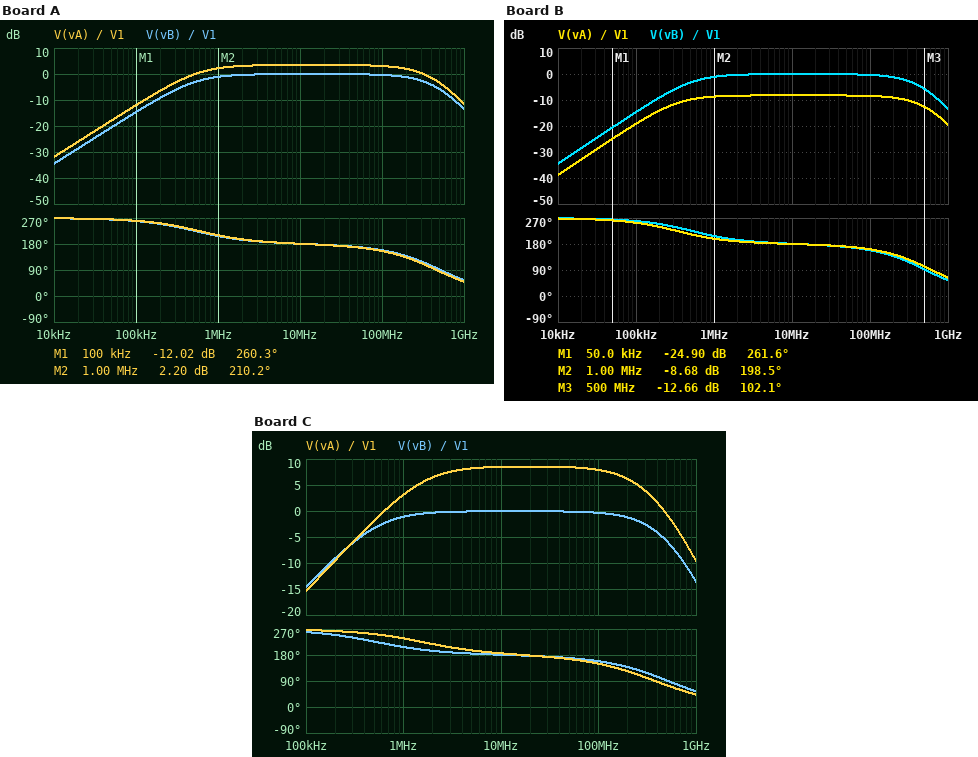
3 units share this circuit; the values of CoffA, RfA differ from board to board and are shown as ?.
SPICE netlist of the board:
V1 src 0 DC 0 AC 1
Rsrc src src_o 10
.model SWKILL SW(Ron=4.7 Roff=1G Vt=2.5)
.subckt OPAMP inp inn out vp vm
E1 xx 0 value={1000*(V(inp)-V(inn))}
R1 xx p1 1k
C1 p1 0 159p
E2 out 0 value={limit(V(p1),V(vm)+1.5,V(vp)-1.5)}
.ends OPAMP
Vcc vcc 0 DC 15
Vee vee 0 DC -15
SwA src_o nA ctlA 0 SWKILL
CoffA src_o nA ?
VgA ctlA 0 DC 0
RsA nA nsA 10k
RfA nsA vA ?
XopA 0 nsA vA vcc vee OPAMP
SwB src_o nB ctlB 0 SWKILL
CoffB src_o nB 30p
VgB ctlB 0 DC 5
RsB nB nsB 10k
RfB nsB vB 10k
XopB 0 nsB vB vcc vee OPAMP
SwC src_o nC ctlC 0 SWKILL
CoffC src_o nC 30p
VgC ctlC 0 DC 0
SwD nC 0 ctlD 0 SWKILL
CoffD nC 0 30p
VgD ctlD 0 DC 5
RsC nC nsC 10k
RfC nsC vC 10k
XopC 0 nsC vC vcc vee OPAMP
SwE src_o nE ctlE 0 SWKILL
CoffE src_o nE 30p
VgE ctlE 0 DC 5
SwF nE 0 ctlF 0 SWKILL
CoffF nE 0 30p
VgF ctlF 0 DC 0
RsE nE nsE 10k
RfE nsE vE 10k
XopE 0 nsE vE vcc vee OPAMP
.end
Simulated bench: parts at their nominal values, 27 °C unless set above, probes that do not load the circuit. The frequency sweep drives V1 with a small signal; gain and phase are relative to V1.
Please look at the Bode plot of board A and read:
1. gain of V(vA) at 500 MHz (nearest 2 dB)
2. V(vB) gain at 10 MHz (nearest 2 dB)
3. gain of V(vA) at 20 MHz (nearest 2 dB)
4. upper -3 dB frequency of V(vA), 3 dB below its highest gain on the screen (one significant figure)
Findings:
-4 dB
0 dB
4 dB
300 MHz
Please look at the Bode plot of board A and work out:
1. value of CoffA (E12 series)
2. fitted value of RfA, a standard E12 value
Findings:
27 pF
15 kΩ
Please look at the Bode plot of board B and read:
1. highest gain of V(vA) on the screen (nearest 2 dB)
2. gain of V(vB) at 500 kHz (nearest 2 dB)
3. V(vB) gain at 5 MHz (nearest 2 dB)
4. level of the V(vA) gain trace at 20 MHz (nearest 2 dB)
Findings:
-8 dB
-4 dB
0 dB
-8 dB
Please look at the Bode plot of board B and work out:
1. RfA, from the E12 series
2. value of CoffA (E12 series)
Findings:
3.9 kΩ
47 pF
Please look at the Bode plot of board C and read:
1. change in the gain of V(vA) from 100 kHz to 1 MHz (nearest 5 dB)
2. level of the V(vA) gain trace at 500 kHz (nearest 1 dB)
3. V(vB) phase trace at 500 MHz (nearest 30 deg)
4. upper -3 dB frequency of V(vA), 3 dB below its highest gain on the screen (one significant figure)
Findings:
20 dB
-2 dB
90 deg
200 MHz
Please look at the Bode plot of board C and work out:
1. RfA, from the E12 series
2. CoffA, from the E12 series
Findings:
27 kΩ
10 pF
